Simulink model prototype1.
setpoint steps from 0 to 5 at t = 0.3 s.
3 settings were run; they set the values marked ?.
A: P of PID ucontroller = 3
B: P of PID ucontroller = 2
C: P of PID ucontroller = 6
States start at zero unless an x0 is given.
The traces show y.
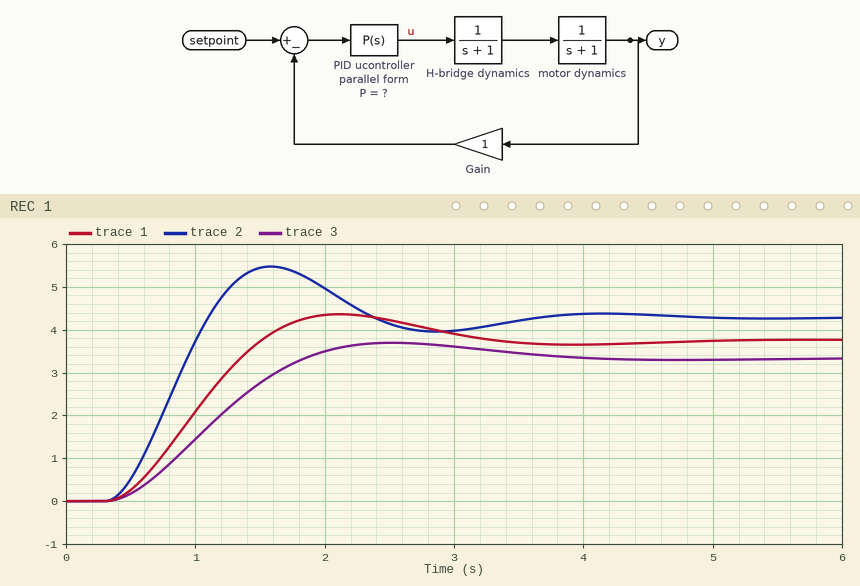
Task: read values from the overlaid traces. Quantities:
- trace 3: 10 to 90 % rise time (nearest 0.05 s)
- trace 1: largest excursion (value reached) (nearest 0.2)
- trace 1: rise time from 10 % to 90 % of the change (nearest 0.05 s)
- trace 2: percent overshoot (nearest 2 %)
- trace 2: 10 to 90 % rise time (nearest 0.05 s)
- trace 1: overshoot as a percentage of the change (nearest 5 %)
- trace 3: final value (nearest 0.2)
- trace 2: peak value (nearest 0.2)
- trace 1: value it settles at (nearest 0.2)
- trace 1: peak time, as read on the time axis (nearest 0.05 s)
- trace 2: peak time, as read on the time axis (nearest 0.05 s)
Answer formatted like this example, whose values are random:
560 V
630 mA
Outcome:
1.05 s
4.4
0.80 s
28 %
0.55 s
15 %
3.4
5.4
3.8
2.10 s
1.60 s
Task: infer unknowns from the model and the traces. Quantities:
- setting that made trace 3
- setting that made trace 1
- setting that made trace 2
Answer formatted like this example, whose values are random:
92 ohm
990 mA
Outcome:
B
A
C
